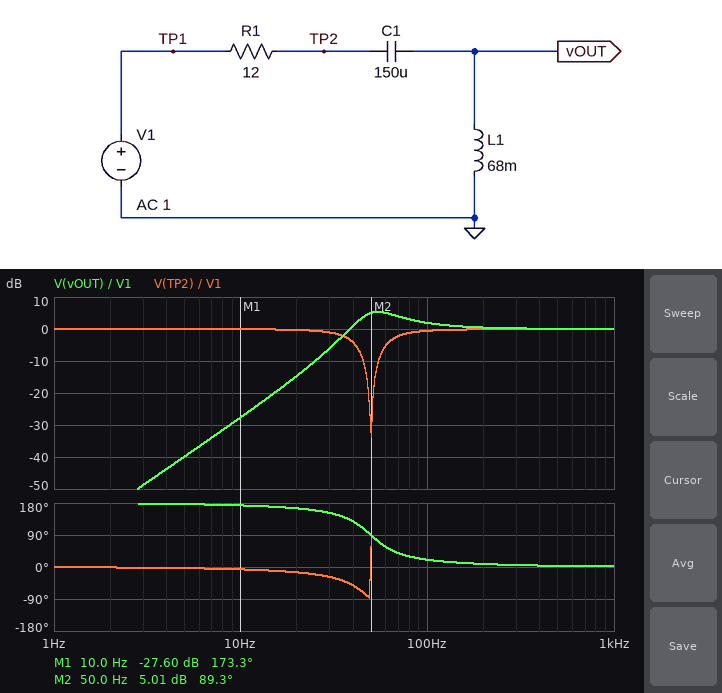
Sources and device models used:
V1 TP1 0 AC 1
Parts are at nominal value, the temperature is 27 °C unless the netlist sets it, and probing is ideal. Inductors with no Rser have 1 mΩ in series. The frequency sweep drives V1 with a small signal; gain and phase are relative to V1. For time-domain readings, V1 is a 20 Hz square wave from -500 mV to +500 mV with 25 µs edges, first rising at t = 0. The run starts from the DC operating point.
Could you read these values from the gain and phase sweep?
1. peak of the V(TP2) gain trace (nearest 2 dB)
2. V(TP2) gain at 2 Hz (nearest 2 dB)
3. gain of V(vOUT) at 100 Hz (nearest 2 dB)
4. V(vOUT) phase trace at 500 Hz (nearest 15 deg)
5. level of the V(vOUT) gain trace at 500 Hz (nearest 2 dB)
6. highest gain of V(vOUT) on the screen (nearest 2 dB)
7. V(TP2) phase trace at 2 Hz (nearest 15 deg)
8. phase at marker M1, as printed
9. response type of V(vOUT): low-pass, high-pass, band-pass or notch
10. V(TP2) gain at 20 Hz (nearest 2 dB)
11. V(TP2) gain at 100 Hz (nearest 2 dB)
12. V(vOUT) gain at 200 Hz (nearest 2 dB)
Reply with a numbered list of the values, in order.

1. 0 dB
2. 0 dB
3. 2 dB
4. 0 deg
5. 0 dB
6. 6 dB
7. 0 deg
8. 173.3 deg
9. high-pass
10. 0 dB
11. 0 dB
12. 0 dB
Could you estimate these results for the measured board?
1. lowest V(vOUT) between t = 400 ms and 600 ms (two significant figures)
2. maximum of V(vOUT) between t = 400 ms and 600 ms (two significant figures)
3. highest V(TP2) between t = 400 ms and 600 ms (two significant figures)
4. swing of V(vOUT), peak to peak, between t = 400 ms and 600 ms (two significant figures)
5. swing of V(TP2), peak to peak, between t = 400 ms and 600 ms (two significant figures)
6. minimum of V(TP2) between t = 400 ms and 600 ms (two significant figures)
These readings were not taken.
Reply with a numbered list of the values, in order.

1. -980 mV
2. 980 mV
3. 640 mV
4. 2.0 V
5. 1.3 V
6. -640 mV
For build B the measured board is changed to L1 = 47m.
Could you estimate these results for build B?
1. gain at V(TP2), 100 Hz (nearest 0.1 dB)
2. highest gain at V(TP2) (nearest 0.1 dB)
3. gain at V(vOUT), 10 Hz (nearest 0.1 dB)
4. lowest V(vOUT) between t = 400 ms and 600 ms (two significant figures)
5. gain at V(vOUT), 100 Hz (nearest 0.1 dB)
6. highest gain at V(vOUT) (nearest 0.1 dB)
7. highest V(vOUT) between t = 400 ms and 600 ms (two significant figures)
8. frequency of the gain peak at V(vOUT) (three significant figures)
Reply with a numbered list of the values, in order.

1. -1.5 dB
2. 0 dB
3. -30.9 dB
4. -1.0 V
5. 2.4 dB
6. 3.9 dB
7. 1.0 V
8. 68.3 Hz
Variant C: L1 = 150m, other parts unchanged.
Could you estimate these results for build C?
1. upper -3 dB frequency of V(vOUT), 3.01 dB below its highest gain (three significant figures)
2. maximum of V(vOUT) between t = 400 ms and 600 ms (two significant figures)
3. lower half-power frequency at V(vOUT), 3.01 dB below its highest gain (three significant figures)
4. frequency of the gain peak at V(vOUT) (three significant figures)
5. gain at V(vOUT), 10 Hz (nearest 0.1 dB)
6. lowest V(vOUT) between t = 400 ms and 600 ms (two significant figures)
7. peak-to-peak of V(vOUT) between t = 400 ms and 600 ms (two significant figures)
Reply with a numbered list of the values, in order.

1. 45.0 Hz
2. 750 mV
3. 29.4 Hz
4. 34.8 Hz
5. -20.3 dB
6. -750 mV
7. 1.5 V
